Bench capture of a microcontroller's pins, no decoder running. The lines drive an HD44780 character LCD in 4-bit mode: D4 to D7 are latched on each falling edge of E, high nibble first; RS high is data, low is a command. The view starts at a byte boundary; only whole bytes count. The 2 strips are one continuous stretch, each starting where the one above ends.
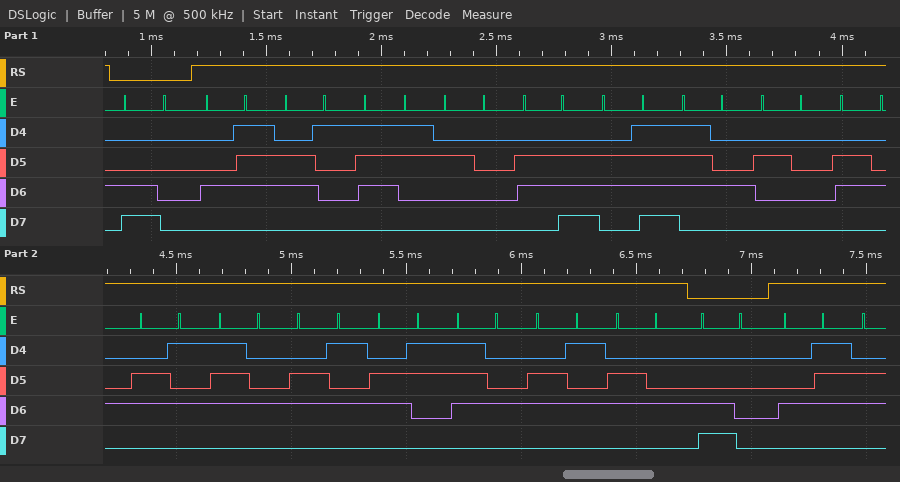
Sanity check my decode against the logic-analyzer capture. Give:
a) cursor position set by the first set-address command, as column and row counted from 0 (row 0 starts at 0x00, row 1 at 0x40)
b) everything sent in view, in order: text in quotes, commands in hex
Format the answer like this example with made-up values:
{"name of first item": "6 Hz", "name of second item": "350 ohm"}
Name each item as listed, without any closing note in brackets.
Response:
{"cursor position set by the first set-address command, as column and row counted from 0": "column 0, row 1", "everything sent in view, in order: text in quotes, commands in hex": "0xC0 \"Gas not detected\" 0xC0 \"G\""}
